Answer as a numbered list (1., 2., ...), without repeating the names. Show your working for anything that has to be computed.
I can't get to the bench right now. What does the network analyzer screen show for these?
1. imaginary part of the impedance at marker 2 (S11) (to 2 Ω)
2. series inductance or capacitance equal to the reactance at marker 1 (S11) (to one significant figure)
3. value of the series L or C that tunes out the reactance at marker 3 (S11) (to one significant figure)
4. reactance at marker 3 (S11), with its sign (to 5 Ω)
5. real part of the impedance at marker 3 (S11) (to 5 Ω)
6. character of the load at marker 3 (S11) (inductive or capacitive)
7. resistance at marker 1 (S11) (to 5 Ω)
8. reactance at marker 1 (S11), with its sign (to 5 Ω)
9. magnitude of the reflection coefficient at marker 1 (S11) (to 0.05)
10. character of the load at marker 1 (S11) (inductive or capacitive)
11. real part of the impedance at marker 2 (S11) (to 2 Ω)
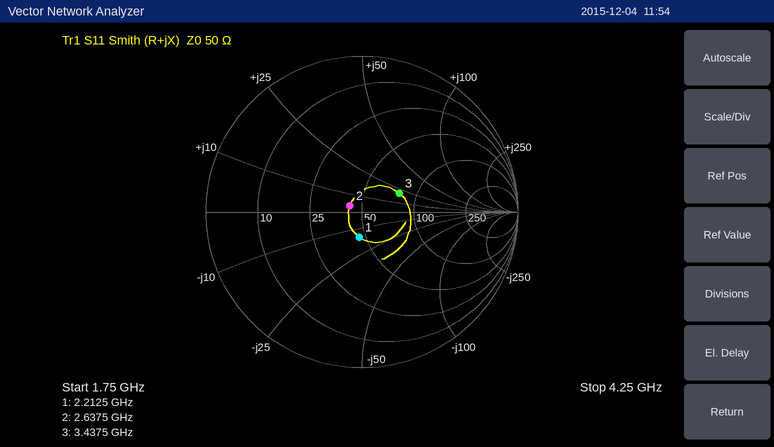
1. +4 Ω
2. C = 1/(2π × 2.2125 GHz × 15 Ω) ≈ 5 pF
3. C = 1/(2π × 3.4375 GHz × 20 Ω) ≈ 2 pF
4. +20 Ω
5. 80 Ω
6. inductive
7. 45 Ω
8. -15 Ω
9. 0.15
10. capacitive
11. 42 Ω
